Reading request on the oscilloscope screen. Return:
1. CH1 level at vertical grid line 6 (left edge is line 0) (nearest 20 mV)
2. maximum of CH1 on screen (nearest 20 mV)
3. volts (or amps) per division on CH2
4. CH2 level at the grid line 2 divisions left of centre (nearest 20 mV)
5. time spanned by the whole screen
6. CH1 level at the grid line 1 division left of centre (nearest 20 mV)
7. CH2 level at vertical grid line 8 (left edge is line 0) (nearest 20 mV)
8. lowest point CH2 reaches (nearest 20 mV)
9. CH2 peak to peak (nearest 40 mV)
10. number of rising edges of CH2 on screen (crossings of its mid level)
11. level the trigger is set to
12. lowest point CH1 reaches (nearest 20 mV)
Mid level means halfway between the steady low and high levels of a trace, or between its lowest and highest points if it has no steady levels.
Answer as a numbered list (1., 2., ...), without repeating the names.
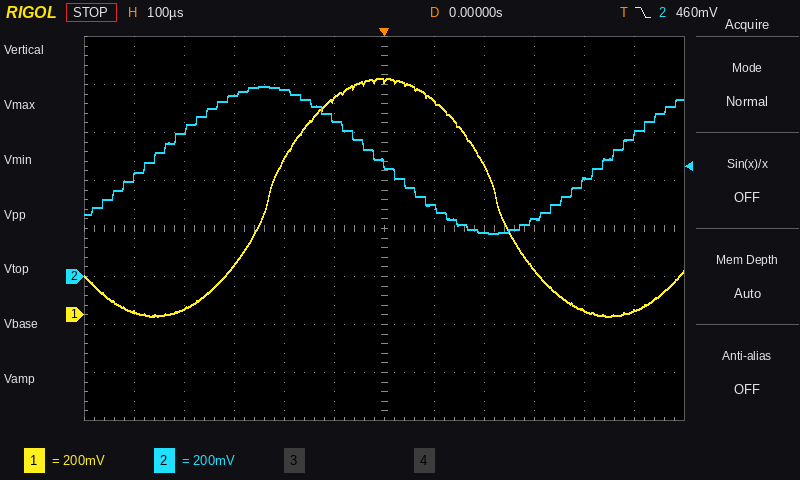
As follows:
1. 980 mV
2. 980 mV
3. 200 mV
4. 780 mV
5. 1.2 ms
6. 900 mV
7. 180 mV
8. 180 mV
9. 600 mV
10. 2
11. 460 mV
12. 0 mV
